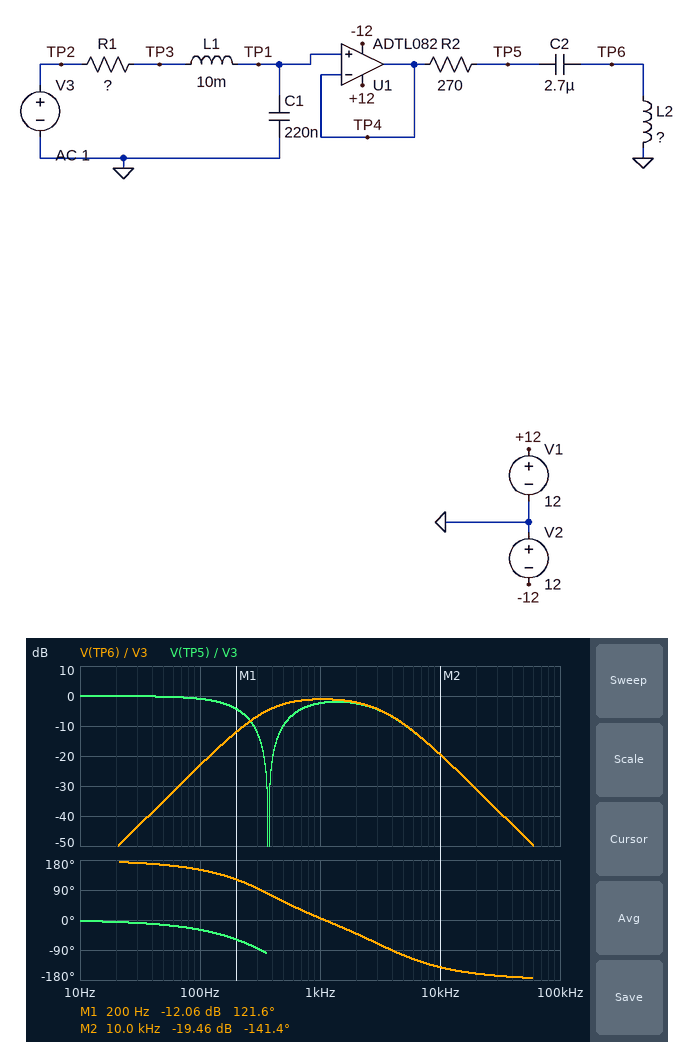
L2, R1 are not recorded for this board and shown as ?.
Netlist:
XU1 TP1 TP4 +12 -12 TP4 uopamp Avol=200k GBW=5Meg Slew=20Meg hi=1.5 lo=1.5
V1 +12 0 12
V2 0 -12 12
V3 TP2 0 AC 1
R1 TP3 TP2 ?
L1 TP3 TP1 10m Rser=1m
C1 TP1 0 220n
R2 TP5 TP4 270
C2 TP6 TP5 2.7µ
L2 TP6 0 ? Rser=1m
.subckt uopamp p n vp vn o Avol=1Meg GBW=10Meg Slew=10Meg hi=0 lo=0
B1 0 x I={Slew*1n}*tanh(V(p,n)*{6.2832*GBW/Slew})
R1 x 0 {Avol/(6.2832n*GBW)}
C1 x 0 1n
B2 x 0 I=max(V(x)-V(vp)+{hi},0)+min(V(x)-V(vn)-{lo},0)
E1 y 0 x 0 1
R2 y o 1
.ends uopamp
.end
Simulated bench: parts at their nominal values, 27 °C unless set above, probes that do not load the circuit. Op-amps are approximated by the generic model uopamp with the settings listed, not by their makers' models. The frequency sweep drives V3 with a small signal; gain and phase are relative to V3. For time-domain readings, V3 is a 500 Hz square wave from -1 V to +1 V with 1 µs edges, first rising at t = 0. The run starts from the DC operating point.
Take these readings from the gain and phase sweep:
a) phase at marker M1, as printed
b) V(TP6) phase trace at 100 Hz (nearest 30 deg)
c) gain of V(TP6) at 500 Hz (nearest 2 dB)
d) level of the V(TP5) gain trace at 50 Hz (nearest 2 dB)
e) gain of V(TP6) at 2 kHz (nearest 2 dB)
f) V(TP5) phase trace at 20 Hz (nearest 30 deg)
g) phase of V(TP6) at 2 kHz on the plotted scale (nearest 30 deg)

121.6 deg
150 deg
-2 dB
0 dB
-2 dB
0 deg
-30 deg
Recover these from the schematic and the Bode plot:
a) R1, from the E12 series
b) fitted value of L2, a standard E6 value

390 Ω
68 mH
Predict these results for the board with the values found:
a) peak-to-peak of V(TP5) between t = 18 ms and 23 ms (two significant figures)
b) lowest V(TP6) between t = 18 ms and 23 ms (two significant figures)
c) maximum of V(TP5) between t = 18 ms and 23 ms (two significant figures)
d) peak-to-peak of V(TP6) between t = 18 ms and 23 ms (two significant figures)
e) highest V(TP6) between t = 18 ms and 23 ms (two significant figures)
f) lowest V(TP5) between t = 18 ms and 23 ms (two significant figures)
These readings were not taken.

1.9 V
-1.5 V
970 mV
3.0 V
1.5 V
-970 mV
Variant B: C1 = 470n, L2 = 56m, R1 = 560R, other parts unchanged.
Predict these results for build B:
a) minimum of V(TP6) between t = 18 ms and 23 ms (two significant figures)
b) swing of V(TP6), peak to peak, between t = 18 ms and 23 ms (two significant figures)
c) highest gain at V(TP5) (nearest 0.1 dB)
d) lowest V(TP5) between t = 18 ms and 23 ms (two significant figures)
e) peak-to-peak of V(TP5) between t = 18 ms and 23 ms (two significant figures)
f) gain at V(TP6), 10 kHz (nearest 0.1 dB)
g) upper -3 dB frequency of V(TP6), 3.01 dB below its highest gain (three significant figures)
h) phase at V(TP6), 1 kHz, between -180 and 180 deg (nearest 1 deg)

-800 mV
1.6 V
0 dB
-380 mV
750 mV
-27.7 dB
1.47 kHz
-21 deg
